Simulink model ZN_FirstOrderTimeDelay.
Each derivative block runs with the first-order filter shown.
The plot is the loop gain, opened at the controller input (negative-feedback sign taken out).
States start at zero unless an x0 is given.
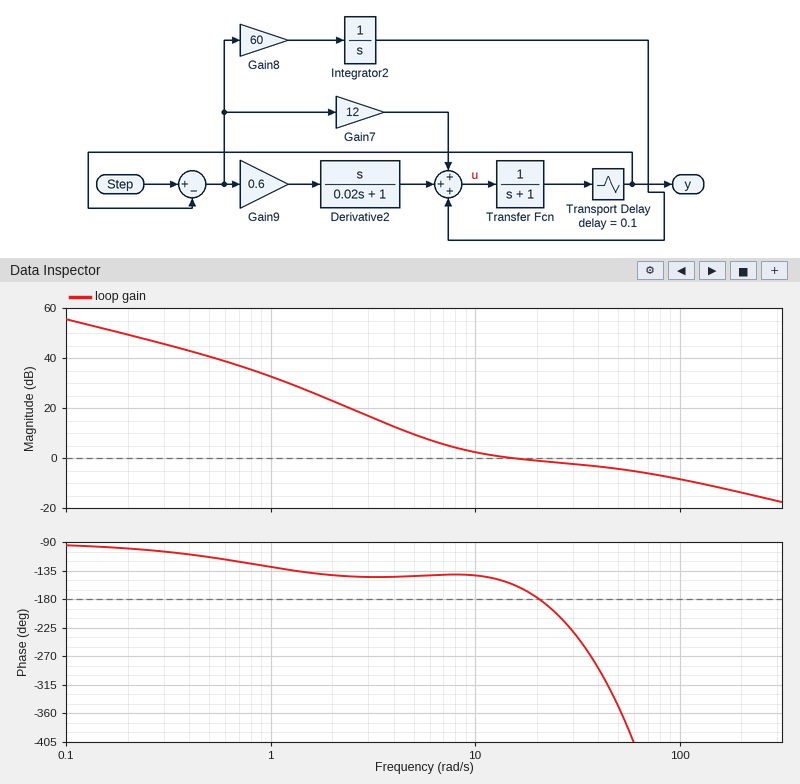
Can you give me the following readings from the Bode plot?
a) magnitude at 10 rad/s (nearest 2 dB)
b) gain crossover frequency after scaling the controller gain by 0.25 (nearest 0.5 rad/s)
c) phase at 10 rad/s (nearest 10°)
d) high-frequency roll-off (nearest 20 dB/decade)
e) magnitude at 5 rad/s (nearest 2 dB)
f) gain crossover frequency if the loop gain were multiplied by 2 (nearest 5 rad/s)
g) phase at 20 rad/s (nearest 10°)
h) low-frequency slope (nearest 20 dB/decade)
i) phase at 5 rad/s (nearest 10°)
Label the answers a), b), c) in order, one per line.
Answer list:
a) 2 dB
b) 4.0 rad/s
c) -140°
d) -20 dB/decade
e) 10 dB
f) 70 rad/s
g) -180°
h) -20 dB/decade
i) -140°
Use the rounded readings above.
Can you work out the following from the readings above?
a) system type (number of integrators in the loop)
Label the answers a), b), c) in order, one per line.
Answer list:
a) 1
